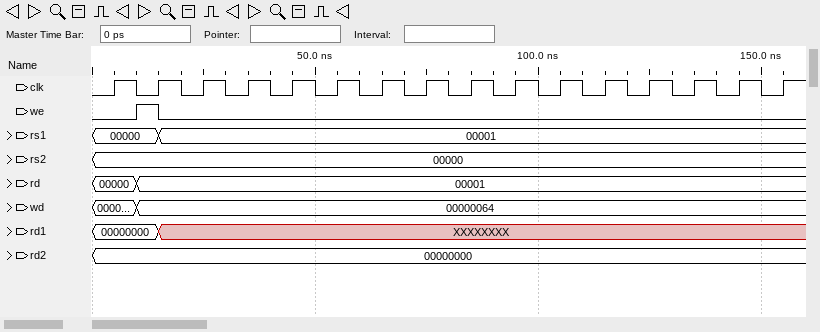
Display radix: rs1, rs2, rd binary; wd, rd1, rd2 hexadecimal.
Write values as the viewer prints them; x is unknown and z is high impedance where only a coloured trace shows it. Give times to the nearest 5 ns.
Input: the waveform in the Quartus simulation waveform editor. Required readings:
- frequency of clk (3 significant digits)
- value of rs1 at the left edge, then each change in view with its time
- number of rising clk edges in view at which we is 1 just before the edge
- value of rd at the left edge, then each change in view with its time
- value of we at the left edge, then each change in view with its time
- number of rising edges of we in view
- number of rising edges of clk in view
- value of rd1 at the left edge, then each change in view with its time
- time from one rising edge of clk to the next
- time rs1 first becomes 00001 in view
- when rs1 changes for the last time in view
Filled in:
100 MHz
00000, 00001 at 15 ns
1
00000, 00001 at 10 ns
0, 1 at 10 ns, 0 at 15 ns
1
16
00000000, XXXXXXXX at 15 ns
10 ns
15 ns
15 ns
